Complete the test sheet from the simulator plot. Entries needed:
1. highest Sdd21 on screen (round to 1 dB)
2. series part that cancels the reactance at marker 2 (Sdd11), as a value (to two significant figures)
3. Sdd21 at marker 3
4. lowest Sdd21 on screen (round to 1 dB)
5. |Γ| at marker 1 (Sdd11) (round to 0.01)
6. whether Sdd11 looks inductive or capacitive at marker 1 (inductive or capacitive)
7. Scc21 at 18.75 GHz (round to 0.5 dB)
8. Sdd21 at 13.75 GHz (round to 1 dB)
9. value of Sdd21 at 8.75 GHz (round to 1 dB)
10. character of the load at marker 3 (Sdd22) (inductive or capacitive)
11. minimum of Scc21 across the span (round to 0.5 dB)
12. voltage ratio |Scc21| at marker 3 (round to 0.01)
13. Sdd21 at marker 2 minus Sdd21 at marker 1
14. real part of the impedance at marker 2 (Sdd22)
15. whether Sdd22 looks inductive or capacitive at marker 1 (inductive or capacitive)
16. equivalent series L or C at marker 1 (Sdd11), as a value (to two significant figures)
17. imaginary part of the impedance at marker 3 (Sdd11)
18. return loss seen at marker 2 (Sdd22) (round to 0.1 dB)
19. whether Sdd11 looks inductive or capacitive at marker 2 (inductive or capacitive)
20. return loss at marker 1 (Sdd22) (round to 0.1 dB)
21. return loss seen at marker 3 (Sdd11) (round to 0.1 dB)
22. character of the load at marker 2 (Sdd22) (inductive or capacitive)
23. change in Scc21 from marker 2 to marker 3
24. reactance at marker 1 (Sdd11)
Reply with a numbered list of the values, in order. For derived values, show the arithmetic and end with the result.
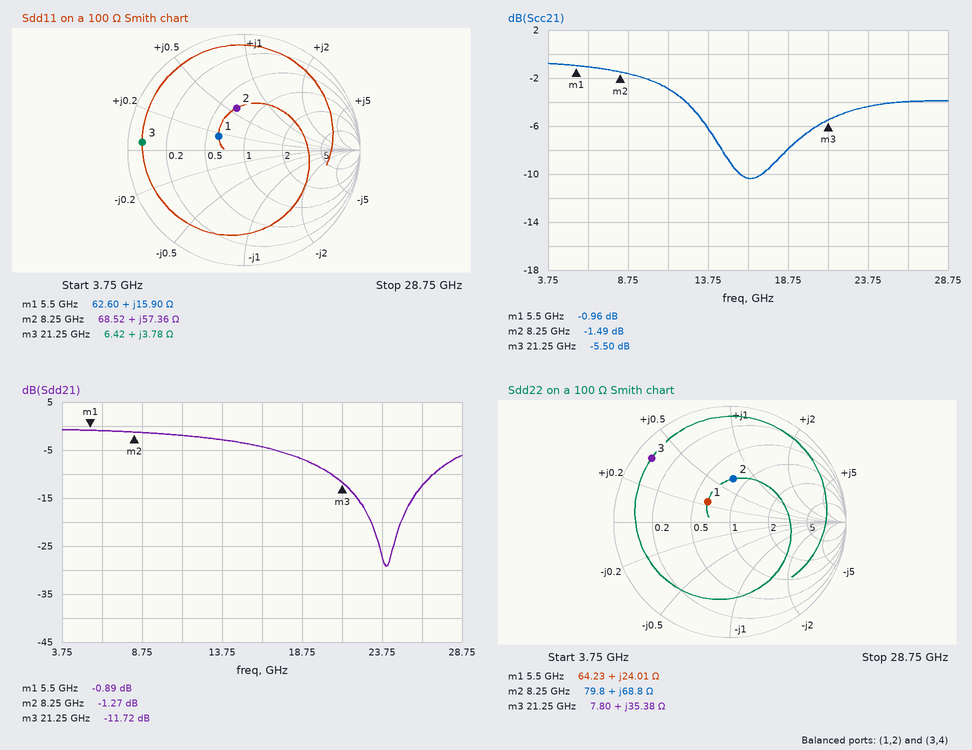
1. -1 dB
2. C = 1/(2π × 8.25 GHz × 57.36 Ω) ≈ 336 fF, so 340 fF to two significant figures
3. -11.72 dB
4. -29 dB
5. 0.25
6. inductive
7. -8.0 dB
8. -3 dB
9. -1 dB
10. inductive
11. -10.5 dB
12. 10^(-5.5/20) ≈ 0.53
13. -1.27 − (-0.89) = -0.38 dB
14. 79.8 Ω
15. inductive
16. L = 15.9 Ω/(2π × 5.5 GHz) ≈ 460 pH
17. +3.78 Ω
18. 8.6 dB
19. inductive
20. 11.7 dB
21. 1.1 dB
22. inductive
23. -5.5 − (-1.49) = -4.01 dB
24. +15.90 Ω
